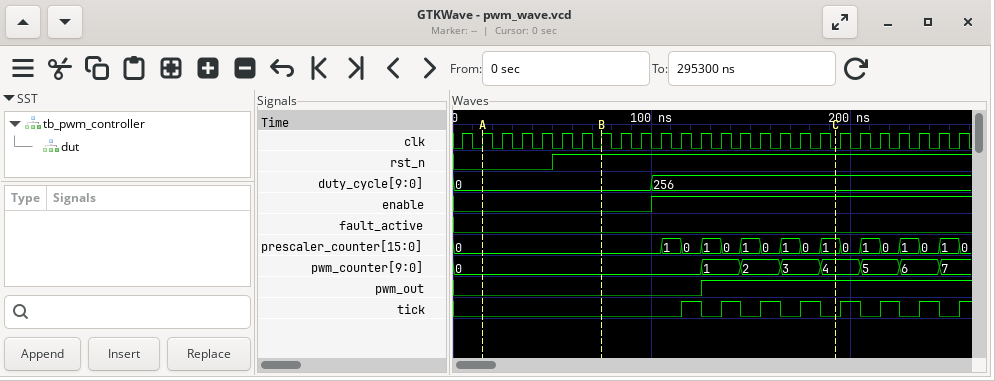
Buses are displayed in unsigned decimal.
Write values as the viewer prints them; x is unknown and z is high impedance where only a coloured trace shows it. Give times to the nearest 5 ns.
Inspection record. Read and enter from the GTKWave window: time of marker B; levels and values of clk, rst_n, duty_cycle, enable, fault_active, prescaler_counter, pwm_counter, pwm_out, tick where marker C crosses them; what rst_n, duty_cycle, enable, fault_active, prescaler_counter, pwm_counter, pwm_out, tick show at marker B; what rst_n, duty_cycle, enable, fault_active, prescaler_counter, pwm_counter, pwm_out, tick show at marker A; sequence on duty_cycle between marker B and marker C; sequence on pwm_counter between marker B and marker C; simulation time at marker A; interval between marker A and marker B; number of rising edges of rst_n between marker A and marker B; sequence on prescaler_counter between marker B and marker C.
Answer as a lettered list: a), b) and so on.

a) 75 ns
b) clk=0, rst_n=1, duty_cycle=256, enable=1, fault_active=0, prescaler_counter=1, pwm_counter=4, pwm_out=1, tick=0
c) rst_n=1, duty_cycle=0, enable=0, fault_active=0, prescaler_counter=0, pwm_counter=0, pwm_out=0, tick=0
d) rst_n=0, duty_cycle=0, enable=0, fault_active=0, prescaler_counter=0, pwm_counter=0, pwm_out=0, tick=0
e) 0, 256
f) 0, 1, 2, 3, 4
g) 15 ns
h) 60 ns
i) 1
j) 0, 1, 0, 1, 0, 1, 0, 1, 0, 1
